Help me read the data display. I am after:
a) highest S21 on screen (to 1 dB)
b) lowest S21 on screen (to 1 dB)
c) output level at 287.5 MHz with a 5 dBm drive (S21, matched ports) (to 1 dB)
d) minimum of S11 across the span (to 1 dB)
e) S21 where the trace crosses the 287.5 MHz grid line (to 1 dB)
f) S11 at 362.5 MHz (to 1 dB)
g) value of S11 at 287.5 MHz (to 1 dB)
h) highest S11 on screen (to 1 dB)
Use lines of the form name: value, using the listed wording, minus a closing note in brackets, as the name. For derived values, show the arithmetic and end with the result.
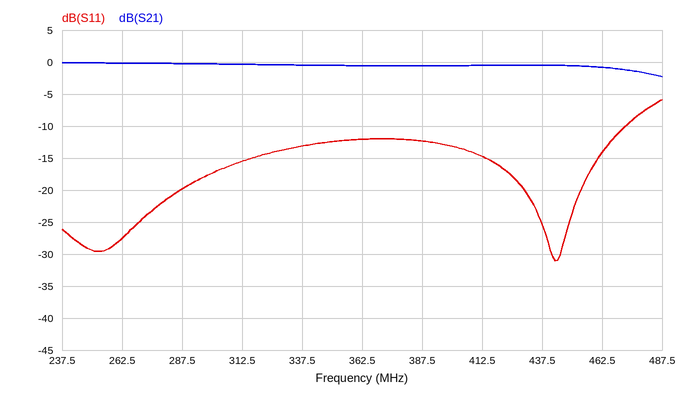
highest S21 on screen: 0 dB
lowest S21 on screen: -2 dB
output level at 287.5 MHz with a 5 dBm drive (S21, matched ports): 5 dBm + (0 dB) = 5 dBm
minimum of S11 across the span: -31 dB
S21 where the trace crosses the 287.5 MHz grid line: 0 dB
S11 at 362.5 MHz: -12 dB
value of S11 at 287.5 MHz: -20 dB
highest S11 on screen: -6 dB
